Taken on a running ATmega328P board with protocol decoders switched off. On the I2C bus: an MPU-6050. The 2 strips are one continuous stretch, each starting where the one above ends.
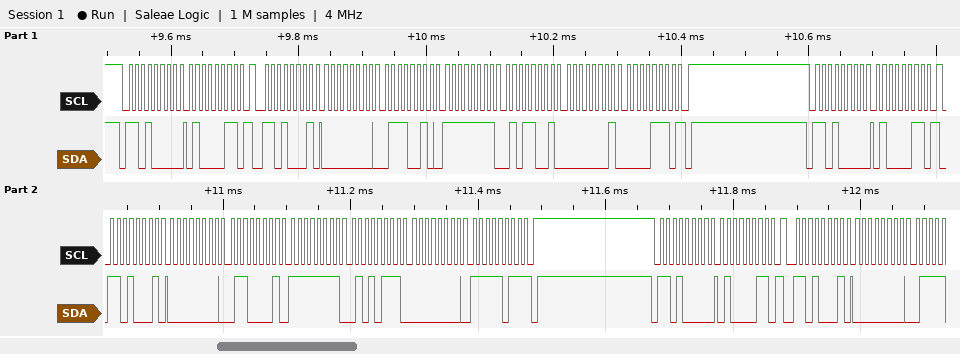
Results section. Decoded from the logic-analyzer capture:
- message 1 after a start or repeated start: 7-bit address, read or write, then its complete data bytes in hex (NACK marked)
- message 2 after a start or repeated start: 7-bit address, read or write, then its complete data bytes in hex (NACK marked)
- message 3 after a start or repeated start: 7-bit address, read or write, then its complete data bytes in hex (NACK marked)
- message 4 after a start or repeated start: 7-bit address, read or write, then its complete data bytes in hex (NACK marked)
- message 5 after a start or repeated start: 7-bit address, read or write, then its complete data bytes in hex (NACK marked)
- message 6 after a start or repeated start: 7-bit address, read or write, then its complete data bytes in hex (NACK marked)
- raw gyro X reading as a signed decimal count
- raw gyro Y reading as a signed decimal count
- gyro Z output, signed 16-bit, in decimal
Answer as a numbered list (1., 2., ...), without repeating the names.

1. 0x68 write: 43
2. 0x68 read: 00 72 FF 59 01 0E NACK
3. 0x68 write: 43
4. 0x68 read: 00 61 FF 57 00 FB NACK
5. 0x68 write: 43
6. 0x68 read: 00
7. 114
8. -167
9. 270
